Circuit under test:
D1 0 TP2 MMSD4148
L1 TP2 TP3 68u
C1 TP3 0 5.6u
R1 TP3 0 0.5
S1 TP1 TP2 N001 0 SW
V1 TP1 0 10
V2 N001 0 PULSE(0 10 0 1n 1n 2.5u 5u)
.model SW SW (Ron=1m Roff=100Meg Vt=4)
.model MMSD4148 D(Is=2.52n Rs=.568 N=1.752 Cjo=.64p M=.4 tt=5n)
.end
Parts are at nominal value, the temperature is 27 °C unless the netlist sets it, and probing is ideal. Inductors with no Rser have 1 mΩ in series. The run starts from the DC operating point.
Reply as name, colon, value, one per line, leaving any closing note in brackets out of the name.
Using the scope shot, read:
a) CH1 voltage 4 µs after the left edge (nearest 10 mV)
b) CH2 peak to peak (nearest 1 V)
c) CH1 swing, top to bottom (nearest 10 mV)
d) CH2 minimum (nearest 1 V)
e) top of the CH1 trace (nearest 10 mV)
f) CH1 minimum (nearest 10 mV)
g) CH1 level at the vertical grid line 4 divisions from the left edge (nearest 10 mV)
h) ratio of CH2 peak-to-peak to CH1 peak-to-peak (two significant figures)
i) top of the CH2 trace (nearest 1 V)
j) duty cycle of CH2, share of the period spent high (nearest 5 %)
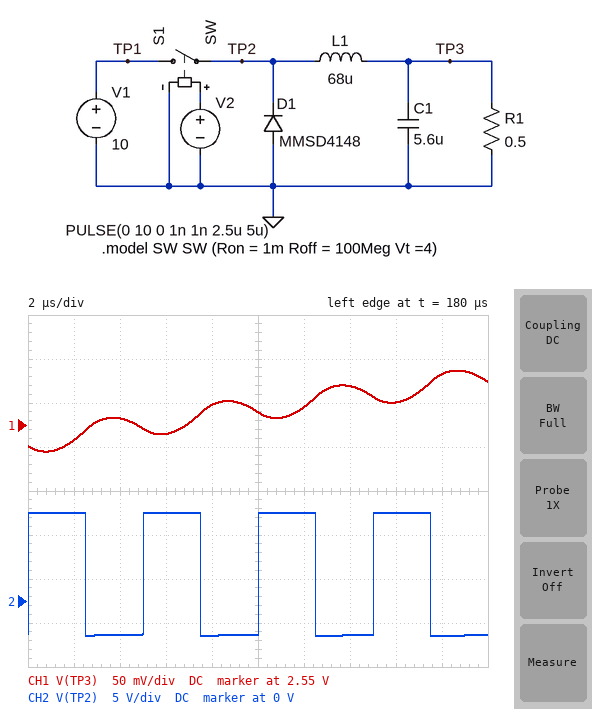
CH1 voltage 4 µs after the left edge: 2.56 V
CH2 peak to peak: 14 V
CH1 swing, top to bottom: 90 mV
CH2 minimum: -4 V
top of the CH1 trace: 2.61 V
CH1 minimum: 2.52 V
CH1 level at the vertical grid line 4 divisions from the left edge: 2.57 V
ratio of CH2 peak-to-peak to CH1 peak-to-peak: 150
top of the CH2 trace: 10 V
duty cycle of CH2, share of the period spent high: 50 %
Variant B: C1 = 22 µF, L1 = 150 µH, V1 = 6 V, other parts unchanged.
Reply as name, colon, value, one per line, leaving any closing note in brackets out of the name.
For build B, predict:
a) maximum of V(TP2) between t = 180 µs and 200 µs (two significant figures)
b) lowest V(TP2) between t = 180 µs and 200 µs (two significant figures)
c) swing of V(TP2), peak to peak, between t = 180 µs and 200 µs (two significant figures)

maximum of V(TP2) between t = 180 µs and 200 µs: 6.0 V
lowest V(TP2) between t = 180 µs and 200 µs: -2.2 V
swing of V(TP2), peak to peak, between t = 180 µs and 200 µs: 8.2 V
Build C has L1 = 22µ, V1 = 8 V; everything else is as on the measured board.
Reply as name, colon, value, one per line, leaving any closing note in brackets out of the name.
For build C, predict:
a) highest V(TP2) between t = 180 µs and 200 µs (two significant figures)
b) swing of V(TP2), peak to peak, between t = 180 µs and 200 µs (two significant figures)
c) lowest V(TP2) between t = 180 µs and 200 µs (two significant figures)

highest V(TP2) between t = 180 µs and 200 µs: 8.0 V
swing of V(TP2), peak to peak, between t = 180 µs and 200 µs: 12 V
lowest V(TP2) between t = 180 µs and 200 µs: -3.7 V
